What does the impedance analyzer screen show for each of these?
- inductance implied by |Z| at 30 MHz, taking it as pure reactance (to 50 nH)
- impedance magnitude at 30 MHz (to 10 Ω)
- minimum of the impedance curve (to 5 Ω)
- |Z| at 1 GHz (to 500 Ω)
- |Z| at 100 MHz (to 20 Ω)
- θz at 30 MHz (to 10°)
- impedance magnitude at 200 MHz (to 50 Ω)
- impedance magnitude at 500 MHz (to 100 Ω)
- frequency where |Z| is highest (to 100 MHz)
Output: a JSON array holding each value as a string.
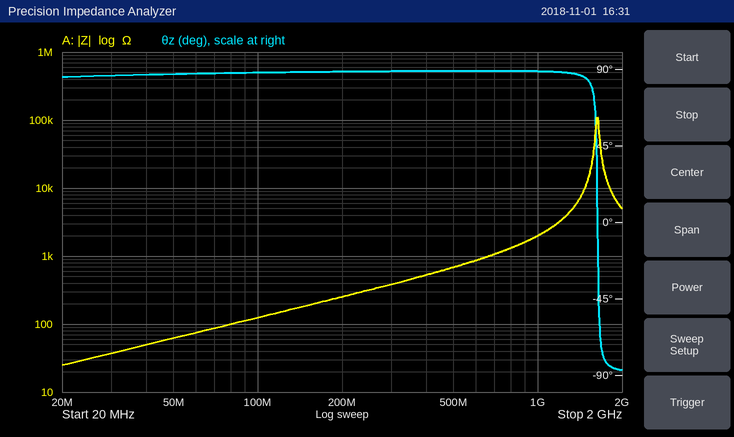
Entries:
["200 nH", "40 Ω", "25 Ω", "2.0 kΩ", "120 Ω", "90°", "250 Ω", "700 Ω", "1.6 GHz"]
